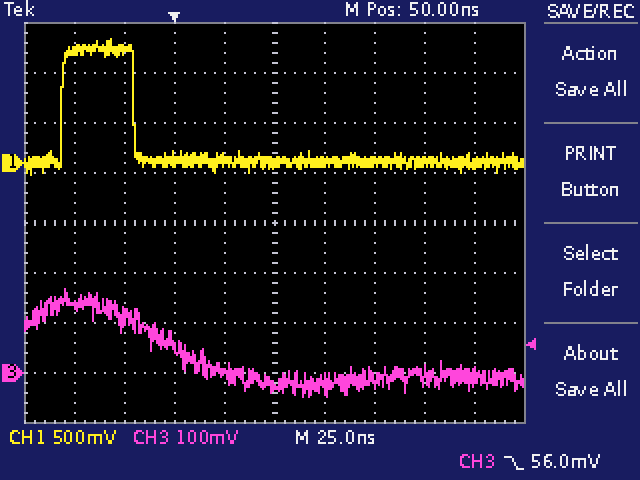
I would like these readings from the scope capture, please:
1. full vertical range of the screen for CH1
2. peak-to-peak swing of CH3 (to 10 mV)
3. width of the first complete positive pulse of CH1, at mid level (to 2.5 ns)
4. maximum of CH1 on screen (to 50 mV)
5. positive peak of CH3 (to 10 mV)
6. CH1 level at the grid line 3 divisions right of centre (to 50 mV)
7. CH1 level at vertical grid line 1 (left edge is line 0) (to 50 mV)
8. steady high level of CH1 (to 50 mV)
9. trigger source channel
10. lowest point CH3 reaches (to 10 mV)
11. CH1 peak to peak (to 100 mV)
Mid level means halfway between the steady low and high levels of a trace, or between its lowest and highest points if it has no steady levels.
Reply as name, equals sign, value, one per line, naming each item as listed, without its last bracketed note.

full vertical range of the screen for CH1 = 4 V
peak-to-peak swing of CH3 = 220 mV
width of the first complete positive pulse of CH1, at mid level = 35.0 ns
maximum of CH1 on screen = 1.25 V
positive peak of CH3 = 170 mV
CH1 level at the grid line 3 divisions right of centre = 0 mV
CH1 level at vertical grid line 1 (left edge is line 0) = 1.15 V
steady high level of CH1 = 1.15 V
trigger source channel = CH3
lowest point CH3 reaches = -50 mV
CH1 peak to peak = 1.40 V
